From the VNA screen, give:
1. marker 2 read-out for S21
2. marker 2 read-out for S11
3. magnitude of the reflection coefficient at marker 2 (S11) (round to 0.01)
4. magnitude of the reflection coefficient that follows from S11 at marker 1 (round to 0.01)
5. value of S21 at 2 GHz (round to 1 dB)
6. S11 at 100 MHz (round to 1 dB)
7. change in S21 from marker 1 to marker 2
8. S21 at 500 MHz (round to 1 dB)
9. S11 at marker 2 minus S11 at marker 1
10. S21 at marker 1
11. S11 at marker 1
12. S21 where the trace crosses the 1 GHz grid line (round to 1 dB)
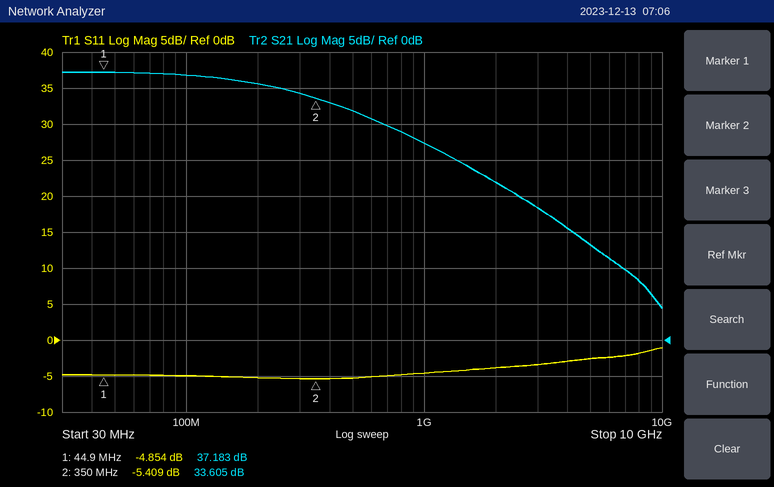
33.605 dB
-5.409 dB
0.54
0.57
22 dB
-5 dB
-3.578 dB
32 dB
-0.555 dB
37.183 dB
-4.854 dB
27 dB
